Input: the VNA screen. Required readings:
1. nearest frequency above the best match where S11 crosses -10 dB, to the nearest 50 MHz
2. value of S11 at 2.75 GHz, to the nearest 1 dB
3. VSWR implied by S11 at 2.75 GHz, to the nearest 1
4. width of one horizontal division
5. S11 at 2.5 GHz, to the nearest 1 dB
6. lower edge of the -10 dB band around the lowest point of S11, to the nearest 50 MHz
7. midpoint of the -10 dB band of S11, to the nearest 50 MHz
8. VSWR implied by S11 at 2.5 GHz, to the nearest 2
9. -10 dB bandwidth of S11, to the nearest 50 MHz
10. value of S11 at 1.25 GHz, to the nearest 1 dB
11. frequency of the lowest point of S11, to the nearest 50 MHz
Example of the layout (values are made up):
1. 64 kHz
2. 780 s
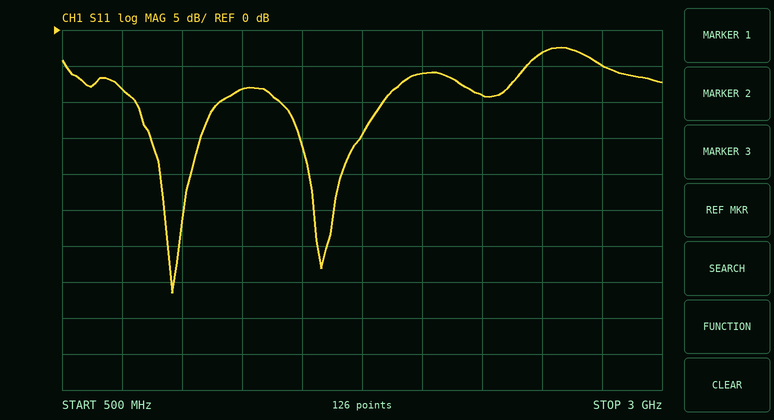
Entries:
1. 1.15 GHz
2. -5 dB
3. 4
4. 250 MHz
5. -3 dB
6. 800 MHz
7. 1.00 GHz
8. 6
9. 350 MHz
10. -8 dB
11. 950 MHz
